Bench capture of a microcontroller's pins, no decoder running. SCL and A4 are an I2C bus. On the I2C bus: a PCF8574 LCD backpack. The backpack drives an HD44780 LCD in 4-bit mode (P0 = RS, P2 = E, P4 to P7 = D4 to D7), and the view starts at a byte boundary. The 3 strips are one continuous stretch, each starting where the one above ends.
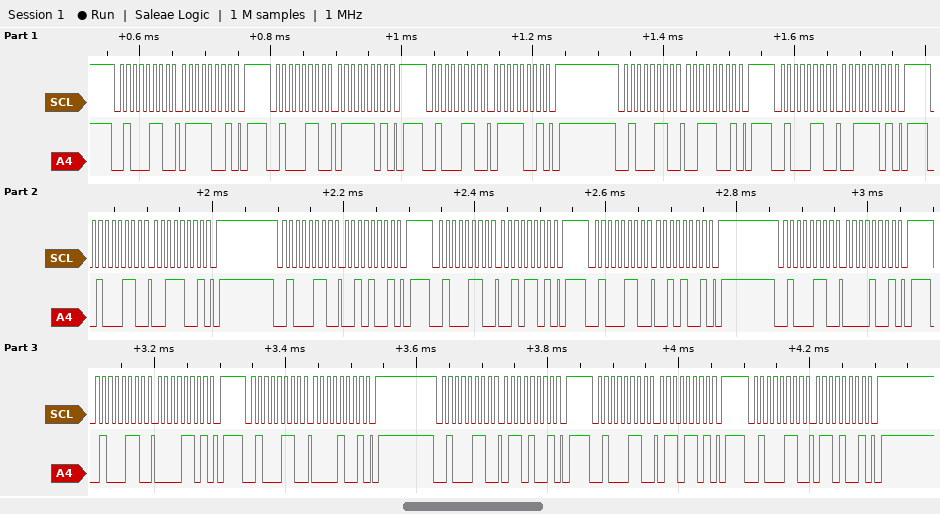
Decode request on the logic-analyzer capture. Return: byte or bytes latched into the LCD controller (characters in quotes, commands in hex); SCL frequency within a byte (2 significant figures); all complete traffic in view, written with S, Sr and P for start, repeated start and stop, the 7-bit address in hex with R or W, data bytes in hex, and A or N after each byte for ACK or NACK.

's' ' '
100 kHz
S 23W A 79 A P S 23W A 7D A P S 23W A 79 A P S 23W A 39 A P S 23W A 3D A P S 23W A 39 A P S 23W A 29 A P S 23W A 2D A P S 23W A 29 A P S 23W A 09 A P S 23W A 0D A P S 23W A 09 A P S 23W A 69 A P S 23W A 6D A P S 23W A 69 A P
